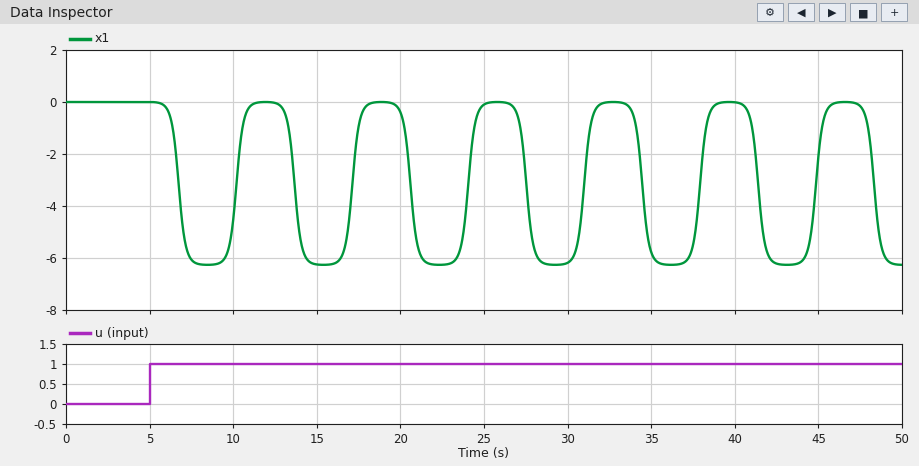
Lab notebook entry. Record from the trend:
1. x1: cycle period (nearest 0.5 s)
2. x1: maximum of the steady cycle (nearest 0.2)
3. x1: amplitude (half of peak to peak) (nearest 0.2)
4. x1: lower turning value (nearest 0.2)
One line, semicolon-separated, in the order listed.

7.0 s; 0.0; 3.2; -6.2
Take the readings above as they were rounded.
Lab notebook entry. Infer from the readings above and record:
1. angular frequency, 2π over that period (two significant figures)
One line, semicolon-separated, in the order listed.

0.90 rad/s
